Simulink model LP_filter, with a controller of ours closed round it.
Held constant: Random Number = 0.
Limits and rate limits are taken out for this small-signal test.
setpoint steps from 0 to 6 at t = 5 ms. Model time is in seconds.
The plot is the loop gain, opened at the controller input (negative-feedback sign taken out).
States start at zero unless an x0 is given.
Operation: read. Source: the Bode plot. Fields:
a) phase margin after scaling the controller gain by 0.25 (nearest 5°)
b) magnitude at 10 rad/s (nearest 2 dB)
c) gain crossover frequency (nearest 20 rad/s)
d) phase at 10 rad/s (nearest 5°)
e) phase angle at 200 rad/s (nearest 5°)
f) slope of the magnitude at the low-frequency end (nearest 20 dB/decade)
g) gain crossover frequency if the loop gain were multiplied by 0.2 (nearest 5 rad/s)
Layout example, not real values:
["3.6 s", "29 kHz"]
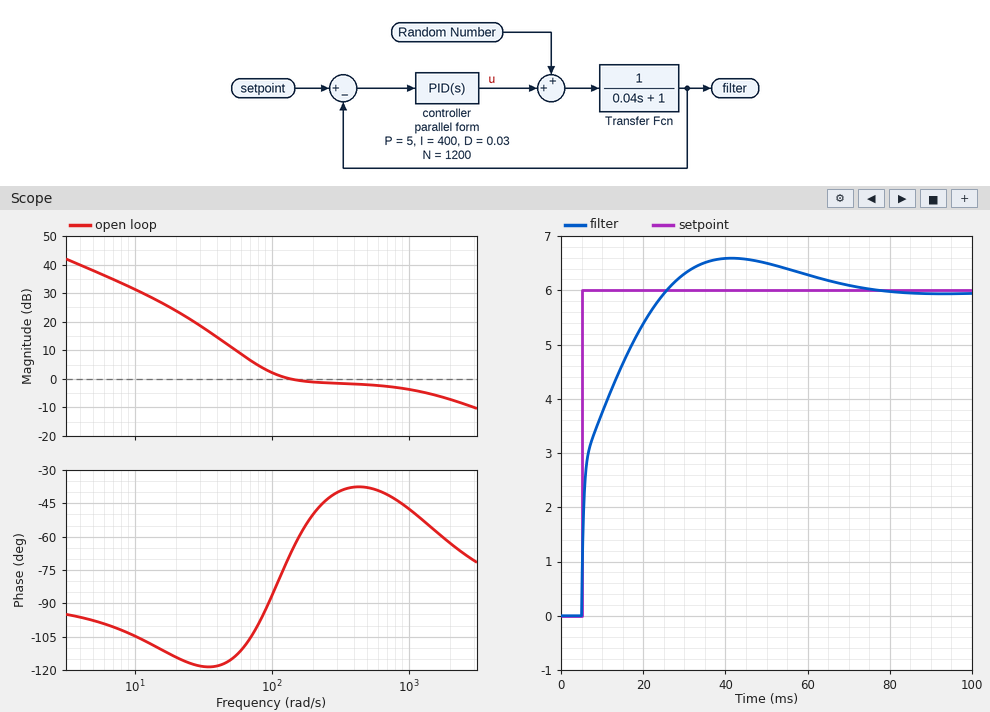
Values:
["65°", "32 dB", "140 rad/s", "-105°", "-50°", "-20 dB/decade", "40 rad/s"]
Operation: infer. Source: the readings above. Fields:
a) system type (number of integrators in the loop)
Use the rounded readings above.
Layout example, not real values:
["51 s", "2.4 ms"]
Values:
["1"]
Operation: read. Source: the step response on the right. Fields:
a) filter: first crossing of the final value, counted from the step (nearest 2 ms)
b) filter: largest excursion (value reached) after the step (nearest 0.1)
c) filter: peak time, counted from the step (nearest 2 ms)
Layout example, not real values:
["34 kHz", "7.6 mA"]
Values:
["20 ms", "6.6", "36 ms"]
